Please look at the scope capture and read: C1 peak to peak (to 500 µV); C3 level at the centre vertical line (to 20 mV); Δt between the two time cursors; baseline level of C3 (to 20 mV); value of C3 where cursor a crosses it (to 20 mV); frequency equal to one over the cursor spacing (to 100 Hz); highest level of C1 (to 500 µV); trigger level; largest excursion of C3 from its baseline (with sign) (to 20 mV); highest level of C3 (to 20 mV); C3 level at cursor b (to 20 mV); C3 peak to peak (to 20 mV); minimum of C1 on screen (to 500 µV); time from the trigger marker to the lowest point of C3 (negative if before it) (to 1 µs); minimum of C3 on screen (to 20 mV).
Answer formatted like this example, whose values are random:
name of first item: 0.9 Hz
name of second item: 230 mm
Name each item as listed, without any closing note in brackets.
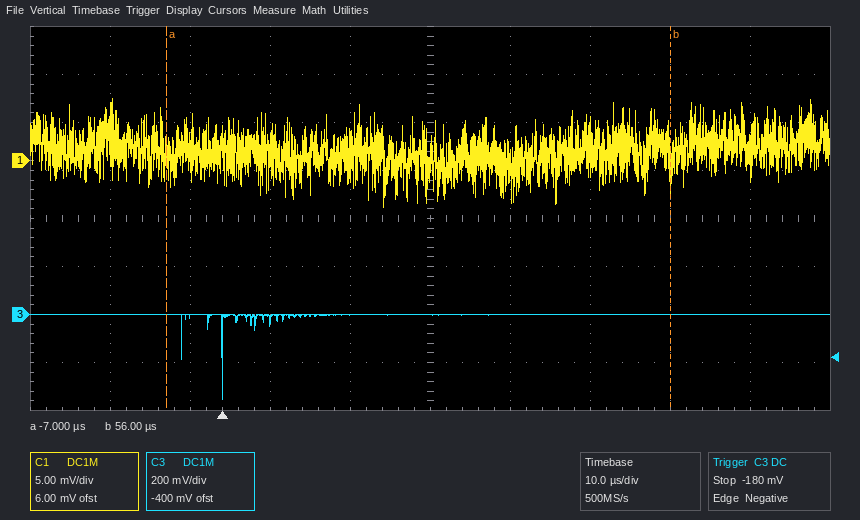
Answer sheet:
C1 peak to peak: 11.5 mV
C3 level at the centre vertical line: 0 mV
Δt between the two time cursors: 63 µs
baseline level of C3: 0 mV
value of C3 where cursor a crosses it: 0 mV
frequency equal to one over the cursor spacing: 15.9 kHz
highest level of C1: 6.5 mV
trigger level: -180 mV
largest excursion of C3 from its baseline (with sign): -360 mV
highest level of C3: 0 mV
C3 level at cursor b: 0 mV
C3 peak to peak: 360 mV
minimum of C1 on screen: -5.0 mV
time from the trigger marker to the lowest point of C3 (negative if before it): 0 µs
minimum of C3 on screen: -360 mV
